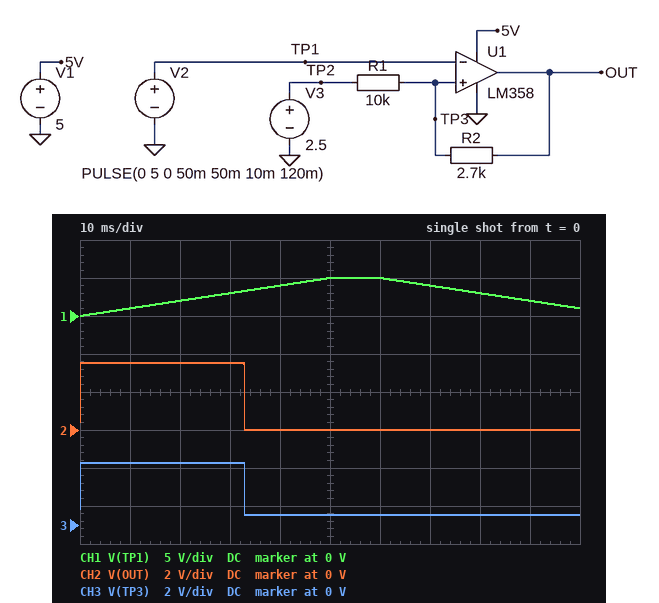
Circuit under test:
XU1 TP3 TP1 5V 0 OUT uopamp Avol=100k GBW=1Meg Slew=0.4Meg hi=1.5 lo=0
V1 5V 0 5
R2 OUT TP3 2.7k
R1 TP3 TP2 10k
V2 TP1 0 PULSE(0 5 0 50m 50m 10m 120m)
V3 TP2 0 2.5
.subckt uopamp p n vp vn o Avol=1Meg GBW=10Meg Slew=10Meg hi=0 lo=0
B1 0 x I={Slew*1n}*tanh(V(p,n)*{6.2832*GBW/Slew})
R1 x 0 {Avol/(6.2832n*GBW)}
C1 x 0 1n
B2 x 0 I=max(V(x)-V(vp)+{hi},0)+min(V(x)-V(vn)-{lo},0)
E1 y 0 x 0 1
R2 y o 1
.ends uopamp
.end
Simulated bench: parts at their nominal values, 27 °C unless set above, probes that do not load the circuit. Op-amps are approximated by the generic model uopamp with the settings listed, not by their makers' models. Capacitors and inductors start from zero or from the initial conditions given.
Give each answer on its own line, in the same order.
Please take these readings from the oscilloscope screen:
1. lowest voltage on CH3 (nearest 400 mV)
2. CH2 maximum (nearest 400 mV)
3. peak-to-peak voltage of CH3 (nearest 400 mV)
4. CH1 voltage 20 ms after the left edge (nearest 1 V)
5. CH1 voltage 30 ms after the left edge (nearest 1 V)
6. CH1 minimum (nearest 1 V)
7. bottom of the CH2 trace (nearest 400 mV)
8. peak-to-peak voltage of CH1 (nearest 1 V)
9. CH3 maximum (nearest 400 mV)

400 mV
3.6 V
2.8 V
2 V
3 V
0 V
0 V
5 V
3.2 V
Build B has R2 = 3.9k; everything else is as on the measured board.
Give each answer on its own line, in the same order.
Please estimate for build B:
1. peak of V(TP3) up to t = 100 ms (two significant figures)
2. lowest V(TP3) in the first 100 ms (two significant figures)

3.2 V
700 mV
